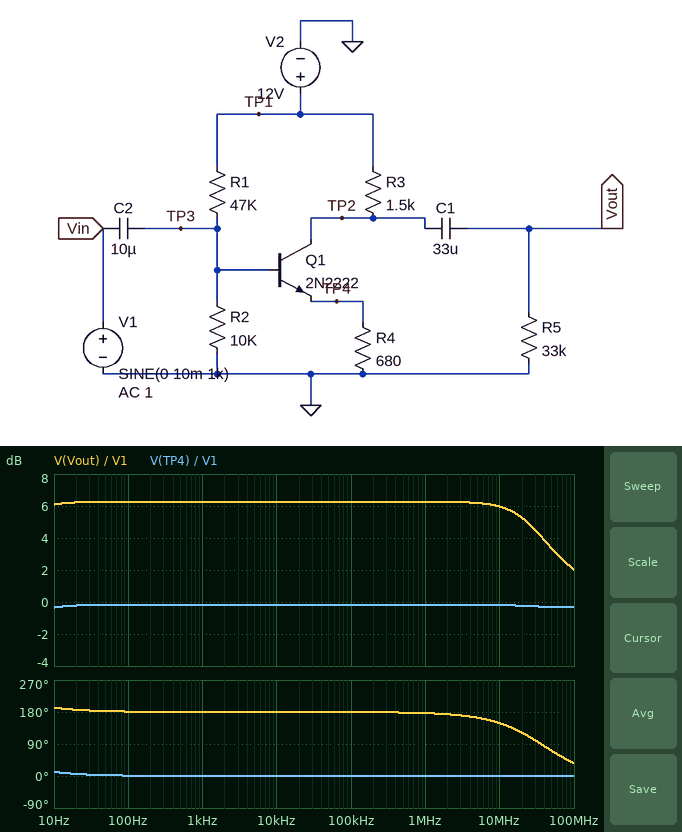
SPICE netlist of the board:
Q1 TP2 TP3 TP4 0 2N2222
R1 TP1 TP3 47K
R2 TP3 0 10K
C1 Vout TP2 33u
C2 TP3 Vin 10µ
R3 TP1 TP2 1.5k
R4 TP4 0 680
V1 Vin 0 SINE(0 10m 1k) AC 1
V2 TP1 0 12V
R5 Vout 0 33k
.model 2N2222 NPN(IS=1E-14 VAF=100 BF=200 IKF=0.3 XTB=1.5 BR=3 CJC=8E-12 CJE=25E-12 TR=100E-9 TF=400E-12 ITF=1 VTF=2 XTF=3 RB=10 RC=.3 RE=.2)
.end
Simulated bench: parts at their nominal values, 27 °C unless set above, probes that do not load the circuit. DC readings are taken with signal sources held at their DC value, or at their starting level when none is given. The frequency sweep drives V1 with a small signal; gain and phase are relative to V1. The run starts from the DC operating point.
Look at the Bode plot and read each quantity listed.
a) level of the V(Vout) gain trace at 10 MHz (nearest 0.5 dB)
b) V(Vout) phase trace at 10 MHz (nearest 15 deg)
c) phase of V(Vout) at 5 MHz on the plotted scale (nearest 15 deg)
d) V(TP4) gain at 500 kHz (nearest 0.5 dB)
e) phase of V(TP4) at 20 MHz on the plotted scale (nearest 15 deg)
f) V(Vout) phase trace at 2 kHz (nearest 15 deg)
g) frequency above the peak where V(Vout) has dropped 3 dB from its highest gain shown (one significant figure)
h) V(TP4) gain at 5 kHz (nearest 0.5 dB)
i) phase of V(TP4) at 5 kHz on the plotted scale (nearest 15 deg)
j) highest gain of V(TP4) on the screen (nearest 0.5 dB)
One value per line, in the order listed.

6.0 dB
150 deg
165 deg
0 dB
0 deg
180 deg
50 MHz
0 dB
0 deg
0 dB
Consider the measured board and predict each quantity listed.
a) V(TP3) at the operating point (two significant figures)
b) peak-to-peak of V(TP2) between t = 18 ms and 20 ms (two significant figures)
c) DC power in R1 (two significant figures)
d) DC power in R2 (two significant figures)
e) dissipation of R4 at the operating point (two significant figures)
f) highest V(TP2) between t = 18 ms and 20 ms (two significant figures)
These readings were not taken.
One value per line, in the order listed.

2.0 V
41 mV
2.1 mW
410 µW
2.7 mW
9.0 V
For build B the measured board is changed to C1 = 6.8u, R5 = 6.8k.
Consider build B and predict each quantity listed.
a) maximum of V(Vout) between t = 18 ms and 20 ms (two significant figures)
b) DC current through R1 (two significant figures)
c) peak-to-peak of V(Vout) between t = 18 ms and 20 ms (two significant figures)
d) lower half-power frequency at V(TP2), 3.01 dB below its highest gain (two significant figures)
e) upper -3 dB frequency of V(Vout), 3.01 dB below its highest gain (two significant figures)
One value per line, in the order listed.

18 mV
210 µA
35 mV
1.5 Hz
98 MHz
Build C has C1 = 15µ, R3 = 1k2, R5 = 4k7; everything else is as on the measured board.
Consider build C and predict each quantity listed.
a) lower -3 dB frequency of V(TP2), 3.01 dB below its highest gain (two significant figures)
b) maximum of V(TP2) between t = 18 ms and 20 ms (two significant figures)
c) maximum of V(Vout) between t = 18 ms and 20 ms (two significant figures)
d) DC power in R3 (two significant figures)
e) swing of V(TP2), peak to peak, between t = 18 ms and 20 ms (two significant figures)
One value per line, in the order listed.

1.6 Hz
9.6 V
14 mV
4.7 mW
27 mV
